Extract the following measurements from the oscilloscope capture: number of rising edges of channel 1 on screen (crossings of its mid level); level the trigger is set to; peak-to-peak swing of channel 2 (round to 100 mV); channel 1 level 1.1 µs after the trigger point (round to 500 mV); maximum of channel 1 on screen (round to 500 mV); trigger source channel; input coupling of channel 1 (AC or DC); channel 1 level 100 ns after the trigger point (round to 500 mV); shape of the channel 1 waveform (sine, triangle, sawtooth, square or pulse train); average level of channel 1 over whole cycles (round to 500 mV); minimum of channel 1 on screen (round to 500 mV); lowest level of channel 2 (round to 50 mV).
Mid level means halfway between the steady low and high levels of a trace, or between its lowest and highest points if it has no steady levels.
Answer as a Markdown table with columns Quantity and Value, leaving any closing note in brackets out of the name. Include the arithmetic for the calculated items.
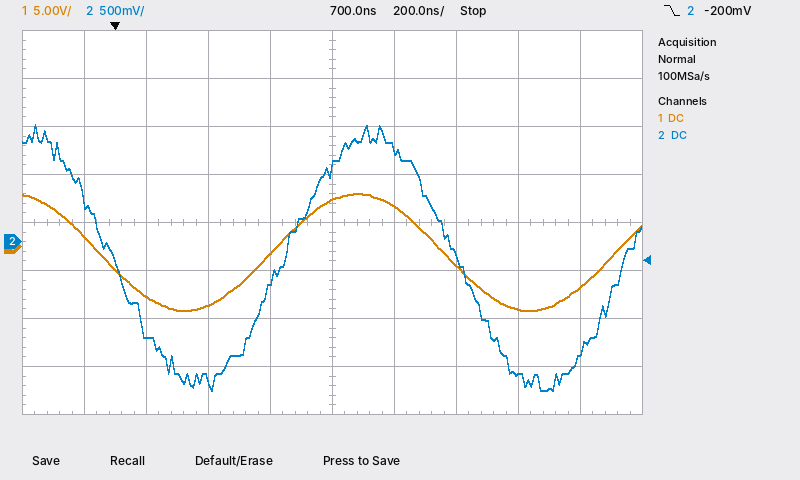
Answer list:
| Quantity | Value |
|---|---|
| number of rising edges of channel 1 on screen | 2 |
| level the trigger is set to | -200 mV |
| peak-to-peak swing of channel 2 | 2.80 V |
| channel 1 level 1.1 µs after the trigger point | -2.0 V |
| maximum of channel 1 on screen | 5.5 V |
| trigger source channel | channel 2 |
| input coupling of channel 1 | DC |
| channel 1 level 100 ns after the trigger point | -5.0 V |
| shape of the channel 1 waveform | sine |
| average level of channel 1 over whole cycles | (5.5 V + (-6.5 V)) / 2 ≈ -500 mV |
| minimum of channel 1 on screen | -6.5 V |
| lowest level of channel 2 | -1.55 V |
